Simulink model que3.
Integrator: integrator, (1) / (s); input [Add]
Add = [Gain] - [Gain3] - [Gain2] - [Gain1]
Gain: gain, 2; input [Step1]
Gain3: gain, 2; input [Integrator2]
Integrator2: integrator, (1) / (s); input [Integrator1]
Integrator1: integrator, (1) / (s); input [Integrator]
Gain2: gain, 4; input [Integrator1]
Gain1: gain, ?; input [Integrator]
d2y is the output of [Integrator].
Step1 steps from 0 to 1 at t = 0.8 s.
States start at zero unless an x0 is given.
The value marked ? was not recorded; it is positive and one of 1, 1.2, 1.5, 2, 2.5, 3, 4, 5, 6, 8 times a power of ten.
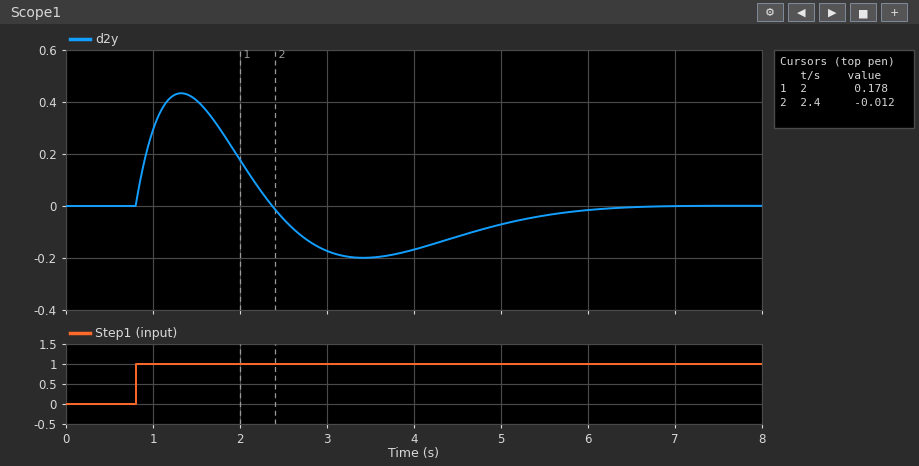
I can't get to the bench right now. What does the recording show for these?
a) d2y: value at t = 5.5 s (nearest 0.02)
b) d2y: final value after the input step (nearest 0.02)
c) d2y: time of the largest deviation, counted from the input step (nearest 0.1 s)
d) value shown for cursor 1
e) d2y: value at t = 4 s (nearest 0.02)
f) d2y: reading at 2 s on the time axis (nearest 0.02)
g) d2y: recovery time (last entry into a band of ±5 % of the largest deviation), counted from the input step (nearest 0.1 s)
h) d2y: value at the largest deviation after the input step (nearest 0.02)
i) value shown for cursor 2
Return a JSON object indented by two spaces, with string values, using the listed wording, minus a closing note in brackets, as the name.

{
  "d2y: value at t = 5.5 s": "-0.04",
  "d2y: final value after the input step": "0.00",
  "d2y: time of the largest deviation, counted from the input step": "0.5 s",
  "value shown for cursor 1": "0.178",
  "d2y: value at t = 4 s": "-0.16",
  "d2y: reading at 2 s on the time axis": "0.18",
  "d2y: recovery time (last entry into a band of ±5 % of the largest deviation), counted from the input step": "5.0 s",
  "d2y: value at the largest deviation after the input step": "0.44",
  "value shown for cursor 2": "-0.012"
}
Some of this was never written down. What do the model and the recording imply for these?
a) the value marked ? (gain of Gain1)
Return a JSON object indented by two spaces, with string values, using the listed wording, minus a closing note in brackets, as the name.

{
  "the value marked ?": "3"
}
